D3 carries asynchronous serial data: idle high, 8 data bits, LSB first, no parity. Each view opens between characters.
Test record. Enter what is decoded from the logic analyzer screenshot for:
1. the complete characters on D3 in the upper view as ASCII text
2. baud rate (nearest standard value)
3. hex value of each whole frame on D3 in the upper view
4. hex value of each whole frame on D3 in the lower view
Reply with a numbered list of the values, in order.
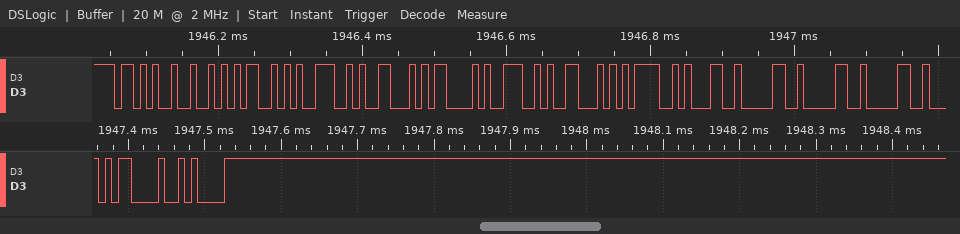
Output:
1. "+RSNFCNF=1000"
2. 115200 baud
3. 2B, 52, 53, 4E, 46, 43, 4E, 46, 3D, 31, 30, 30, 30
4. 0D, 0A
